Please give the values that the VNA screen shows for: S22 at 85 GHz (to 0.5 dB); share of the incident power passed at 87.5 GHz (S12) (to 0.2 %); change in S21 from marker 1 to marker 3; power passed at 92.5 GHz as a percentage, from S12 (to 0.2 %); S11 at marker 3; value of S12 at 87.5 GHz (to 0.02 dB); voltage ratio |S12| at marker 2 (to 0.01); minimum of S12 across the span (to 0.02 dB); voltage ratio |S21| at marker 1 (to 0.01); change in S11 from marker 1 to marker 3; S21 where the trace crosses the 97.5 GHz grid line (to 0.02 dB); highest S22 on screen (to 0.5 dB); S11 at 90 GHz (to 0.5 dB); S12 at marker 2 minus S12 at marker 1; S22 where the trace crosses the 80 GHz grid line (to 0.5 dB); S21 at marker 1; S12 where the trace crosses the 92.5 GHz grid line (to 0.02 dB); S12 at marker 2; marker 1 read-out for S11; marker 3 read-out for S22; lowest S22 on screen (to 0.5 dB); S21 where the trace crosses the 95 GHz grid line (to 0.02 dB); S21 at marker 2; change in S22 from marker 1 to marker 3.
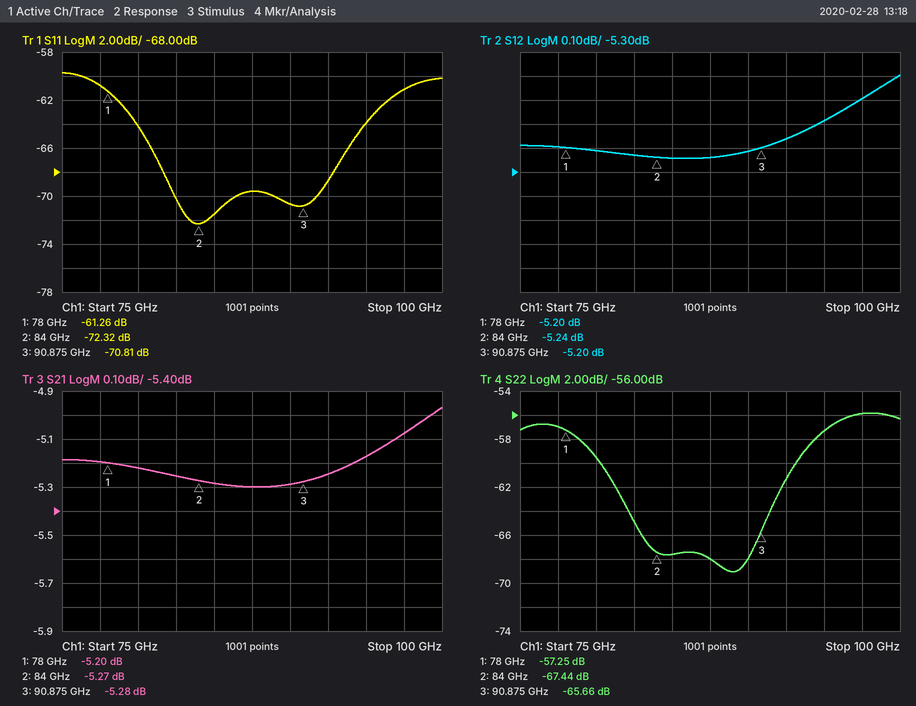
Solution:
-67.5 dB
30.0 %
-0.08 dB
30.4 %
-70.81 dB
-5.24 dB
0.55
-5.24 dB
0.55
-9.55 dB
-5.08 dB
-56.0 dB
-70.5 dB
-0.04 dB
-59.5 dB
-5.20 dB
-5.16 dB
-5.24 dB
-61.26 dB
-65.66 dB
-69.0 dB
-5.18 dB
-5.27 dB
-8.41 dB
